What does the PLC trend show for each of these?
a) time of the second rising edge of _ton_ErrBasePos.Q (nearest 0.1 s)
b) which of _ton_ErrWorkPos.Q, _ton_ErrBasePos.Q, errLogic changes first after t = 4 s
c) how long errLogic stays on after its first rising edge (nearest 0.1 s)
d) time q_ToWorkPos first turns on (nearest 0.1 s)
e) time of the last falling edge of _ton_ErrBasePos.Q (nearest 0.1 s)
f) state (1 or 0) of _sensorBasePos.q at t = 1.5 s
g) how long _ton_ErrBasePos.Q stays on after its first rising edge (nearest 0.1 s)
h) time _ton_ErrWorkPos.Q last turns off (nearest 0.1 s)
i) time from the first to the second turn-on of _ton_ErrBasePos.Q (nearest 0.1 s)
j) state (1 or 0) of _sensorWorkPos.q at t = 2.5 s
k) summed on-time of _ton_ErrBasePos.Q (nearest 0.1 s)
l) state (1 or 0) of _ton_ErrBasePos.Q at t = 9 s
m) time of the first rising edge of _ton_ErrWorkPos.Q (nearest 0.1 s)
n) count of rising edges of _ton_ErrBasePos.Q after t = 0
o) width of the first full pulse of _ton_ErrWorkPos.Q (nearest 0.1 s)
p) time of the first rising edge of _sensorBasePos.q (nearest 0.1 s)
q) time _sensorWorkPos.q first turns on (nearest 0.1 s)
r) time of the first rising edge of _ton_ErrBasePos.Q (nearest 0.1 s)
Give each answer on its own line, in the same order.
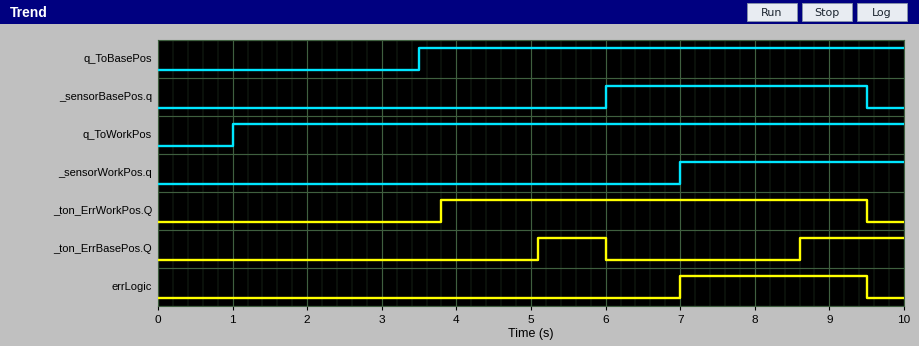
8.6 s
_ton_ErrBasePos.Q
2.5 s
1.0 s
6.0 s
0
0.9 s
9.5 s
3.5 s
0
2.3 s
1
3.8 s
2
5.7 s
6.0 s
7.0 s
5.1 s
